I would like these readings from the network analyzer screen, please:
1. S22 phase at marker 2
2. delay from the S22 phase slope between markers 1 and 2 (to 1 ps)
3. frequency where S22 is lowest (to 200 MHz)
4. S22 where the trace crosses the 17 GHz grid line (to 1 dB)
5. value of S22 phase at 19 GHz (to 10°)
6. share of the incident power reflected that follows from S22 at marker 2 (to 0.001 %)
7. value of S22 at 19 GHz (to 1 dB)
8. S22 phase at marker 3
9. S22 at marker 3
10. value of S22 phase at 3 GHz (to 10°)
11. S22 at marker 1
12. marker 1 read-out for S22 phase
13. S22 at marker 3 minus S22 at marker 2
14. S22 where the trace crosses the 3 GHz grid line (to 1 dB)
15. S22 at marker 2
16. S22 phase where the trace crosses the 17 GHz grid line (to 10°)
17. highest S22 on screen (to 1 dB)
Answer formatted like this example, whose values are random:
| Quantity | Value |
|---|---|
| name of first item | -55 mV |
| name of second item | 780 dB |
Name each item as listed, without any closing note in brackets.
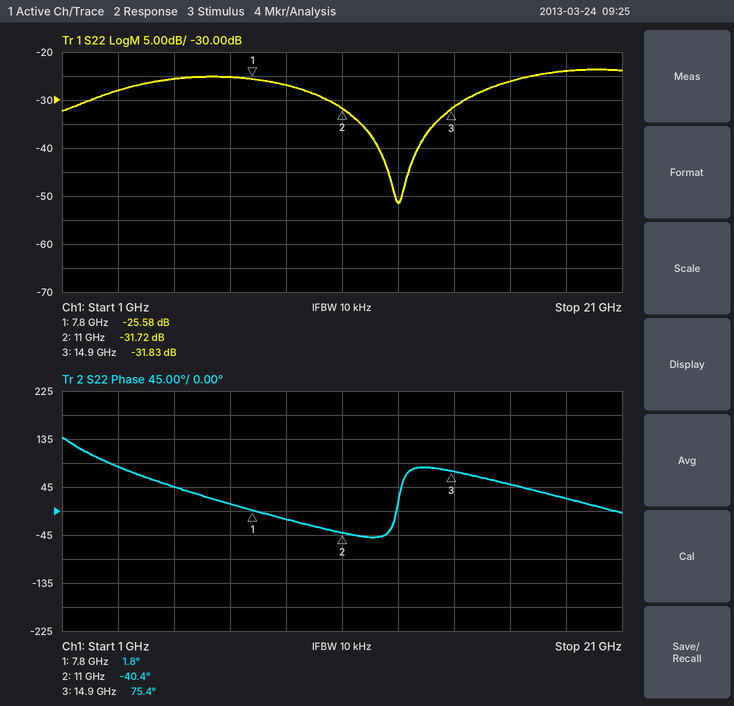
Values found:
| Quantity | Value |
|---|---|
| S22 phase at marker 2 | -40.4° |
| delay from the S22 phase slope between markers 1 and 2 | 37 ps |
| frequency where S22 is lowest | 13.0 GHz |
| S22 where the trace crosses the 17 GHz grid line | -26 dB |
| value of S22 phase at 19 GHz | 20° |
| share of the incident power reflected that follows from S22 at marker 2 | 0.067 % |
| value of S22 at 19 GHz | -24 dB |
| S22 phase at marker 3 | 75.4° |
| S22 at marker 3 | -31.83 dB |
| value of S22 phase at 3 GHz | 80° |
| S22 at marker 1 | -25.58 dB |
| marker 1 read-out for S22 phase | 1.8° |
| S22 at marker 3 minus S22 at marker 2 | -0.11 dB |
| S22 where the trace crosses the 3 GHz grid line | -28 dB |
| S22 at marker 2 | -31.72 dB |
| S22 phase where the trace crosses the 17 GHz grid line | 50° |
| highest S22 on screen | -24 dB |
